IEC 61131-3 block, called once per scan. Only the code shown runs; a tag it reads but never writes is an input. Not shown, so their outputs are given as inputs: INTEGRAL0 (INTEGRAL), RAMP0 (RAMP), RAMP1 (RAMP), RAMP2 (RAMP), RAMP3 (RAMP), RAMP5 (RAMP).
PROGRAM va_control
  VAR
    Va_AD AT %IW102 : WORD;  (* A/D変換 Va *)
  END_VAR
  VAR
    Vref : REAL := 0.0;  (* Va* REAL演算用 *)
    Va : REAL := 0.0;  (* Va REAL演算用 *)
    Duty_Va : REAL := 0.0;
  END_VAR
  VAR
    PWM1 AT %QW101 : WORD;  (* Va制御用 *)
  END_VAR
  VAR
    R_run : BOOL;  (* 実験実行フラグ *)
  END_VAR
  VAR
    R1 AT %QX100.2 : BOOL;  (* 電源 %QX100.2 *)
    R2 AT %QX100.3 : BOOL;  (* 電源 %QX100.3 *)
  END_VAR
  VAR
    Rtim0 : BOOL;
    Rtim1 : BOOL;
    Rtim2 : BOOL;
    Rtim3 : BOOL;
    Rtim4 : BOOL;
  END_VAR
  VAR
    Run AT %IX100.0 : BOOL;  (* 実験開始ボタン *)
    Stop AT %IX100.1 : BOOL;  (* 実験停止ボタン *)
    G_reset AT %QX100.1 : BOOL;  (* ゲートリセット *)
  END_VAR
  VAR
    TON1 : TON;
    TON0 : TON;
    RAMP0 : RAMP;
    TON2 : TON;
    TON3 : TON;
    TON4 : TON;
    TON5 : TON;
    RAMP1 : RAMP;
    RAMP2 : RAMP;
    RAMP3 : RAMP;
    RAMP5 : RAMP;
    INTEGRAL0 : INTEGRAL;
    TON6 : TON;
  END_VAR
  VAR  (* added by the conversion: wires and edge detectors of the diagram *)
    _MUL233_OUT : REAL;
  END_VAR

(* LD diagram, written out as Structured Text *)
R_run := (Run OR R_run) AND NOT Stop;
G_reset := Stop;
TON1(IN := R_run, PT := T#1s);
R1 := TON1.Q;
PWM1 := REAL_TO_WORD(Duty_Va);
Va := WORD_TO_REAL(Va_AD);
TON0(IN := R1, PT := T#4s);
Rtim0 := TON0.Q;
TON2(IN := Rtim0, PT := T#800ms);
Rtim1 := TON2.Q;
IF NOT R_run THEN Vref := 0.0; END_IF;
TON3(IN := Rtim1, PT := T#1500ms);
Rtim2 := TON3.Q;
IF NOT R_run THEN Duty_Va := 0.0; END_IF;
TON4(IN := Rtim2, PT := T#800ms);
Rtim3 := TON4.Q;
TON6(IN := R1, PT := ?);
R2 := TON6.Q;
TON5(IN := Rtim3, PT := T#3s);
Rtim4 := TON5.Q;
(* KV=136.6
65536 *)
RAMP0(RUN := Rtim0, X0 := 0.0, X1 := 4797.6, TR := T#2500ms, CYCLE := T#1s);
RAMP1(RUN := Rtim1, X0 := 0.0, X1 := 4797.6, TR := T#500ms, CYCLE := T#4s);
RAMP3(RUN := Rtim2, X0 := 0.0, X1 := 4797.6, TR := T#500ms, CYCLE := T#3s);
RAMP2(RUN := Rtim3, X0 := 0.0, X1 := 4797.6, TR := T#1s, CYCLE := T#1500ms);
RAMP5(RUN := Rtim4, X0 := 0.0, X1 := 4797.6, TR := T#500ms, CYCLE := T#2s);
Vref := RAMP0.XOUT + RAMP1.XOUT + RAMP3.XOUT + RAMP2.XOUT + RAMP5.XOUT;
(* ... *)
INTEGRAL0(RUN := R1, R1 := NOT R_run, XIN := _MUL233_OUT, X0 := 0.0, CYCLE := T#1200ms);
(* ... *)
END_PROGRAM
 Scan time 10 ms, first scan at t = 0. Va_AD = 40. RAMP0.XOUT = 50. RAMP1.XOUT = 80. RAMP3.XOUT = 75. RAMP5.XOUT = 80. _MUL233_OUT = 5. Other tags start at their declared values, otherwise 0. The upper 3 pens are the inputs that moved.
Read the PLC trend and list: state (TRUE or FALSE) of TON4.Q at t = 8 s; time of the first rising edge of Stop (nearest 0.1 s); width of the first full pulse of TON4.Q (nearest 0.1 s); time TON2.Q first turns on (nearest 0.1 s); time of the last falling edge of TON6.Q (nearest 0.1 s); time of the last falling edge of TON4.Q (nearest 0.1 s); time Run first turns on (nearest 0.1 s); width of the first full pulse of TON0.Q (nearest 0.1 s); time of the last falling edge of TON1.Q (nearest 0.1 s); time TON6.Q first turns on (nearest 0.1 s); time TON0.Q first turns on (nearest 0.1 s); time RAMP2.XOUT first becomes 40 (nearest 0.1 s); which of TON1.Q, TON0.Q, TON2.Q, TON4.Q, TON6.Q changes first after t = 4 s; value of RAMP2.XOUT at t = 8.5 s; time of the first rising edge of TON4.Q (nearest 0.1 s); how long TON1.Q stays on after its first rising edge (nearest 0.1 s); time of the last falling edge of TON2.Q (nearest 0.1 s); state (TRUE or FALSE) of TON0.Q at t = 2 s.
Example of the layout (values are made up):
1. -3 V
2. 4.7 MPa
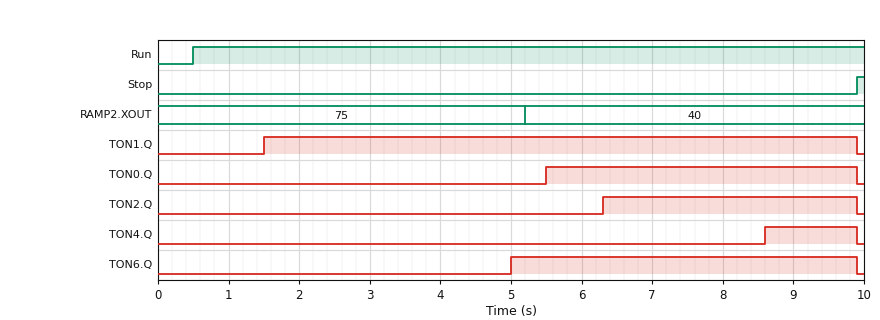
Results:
1. FALSE
2. 9.9 s
3. 1.3 s
4. 6.3 s
5. 9.9 s
6. 9.9 s
7. 0.5 s
8. 4.4 s
9. 9.9 s
10. 5.0 s
11. 5.5 s
12. 5.2 s
13. TON6.Q
14. 40
15. 8.6 s
16. 8.4 s
17. 9.9 s
18. FALSE
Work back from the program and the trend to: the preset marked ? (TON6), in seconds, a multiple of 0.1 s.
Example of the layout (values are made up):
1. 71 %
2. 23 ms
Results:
1. 3.5 s
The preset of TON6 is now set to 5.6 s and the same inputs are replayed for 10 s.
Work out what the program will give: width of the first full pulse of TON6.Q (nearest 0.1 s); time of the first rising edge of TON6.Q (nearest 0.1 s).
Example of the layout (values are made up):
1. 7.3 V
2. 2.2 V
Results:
1. 2.8 s
2. 7.1 s
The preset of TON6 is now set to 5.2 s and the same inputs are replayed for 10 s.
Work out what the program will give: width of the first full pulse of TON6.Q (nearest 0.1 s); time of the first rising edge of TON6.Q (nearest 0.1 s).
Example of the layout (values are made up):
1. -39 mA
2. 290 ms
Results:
1. 3.2 s
2. 6.7 s
